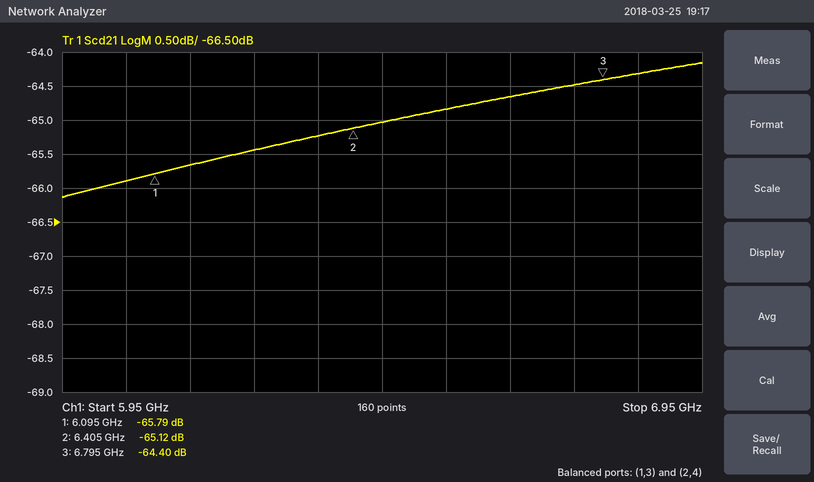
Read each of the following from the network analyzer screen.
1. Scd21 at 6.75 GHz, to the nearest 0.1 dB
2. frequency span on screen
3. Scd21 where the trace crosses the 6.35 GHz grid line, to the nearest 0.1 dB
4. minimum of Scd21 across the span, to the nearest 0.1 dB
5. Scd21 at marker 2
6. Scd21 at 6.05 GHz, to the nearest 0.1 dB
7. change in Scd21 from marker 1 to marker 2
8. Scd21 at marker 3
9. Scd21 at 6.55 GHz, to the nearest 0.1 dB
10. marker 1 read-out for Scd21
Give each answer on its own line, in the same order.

-64.5 dB
1 GHz
-65.2 dB
-66.1 dB
-65.12 dB
-65.9 dB
0.67 dB
-64.40 dB
-64.8 dB
-65.79 dB
